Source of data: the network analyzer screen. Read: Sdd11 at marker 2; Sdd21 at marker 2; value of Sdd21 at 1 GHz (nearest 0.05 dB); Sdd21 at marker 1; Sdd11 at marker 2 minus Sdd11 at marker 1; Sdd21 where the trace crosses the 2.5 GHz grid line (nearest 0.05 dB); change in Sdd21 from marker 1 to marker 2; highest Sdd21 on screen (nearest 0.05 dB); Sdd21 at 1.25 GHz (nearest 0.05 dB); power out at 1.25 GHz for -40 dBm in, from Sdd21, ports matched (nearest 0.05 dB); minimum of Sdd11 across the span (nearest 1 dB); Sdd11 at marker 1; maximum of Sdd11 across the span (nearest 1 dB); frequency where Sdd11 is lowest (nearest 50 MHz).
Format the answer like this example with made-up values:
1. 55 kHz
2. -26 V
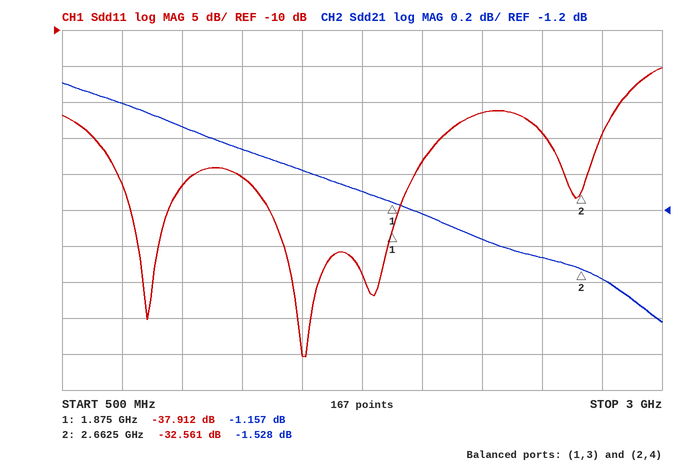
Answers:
1. -32.561 dB
2. -1.528 dB
3. -0.75 dB
4. -1.157 dB
5. 5.351 dB
6. -1.45 dB
7. -0.371 dB
8. -0.50 dB
9. -0.85 dB
10. -40.85 dBm
11. -55 dB
12. -37.912 dB
13. -15 dB
14. 1.50 GHz
